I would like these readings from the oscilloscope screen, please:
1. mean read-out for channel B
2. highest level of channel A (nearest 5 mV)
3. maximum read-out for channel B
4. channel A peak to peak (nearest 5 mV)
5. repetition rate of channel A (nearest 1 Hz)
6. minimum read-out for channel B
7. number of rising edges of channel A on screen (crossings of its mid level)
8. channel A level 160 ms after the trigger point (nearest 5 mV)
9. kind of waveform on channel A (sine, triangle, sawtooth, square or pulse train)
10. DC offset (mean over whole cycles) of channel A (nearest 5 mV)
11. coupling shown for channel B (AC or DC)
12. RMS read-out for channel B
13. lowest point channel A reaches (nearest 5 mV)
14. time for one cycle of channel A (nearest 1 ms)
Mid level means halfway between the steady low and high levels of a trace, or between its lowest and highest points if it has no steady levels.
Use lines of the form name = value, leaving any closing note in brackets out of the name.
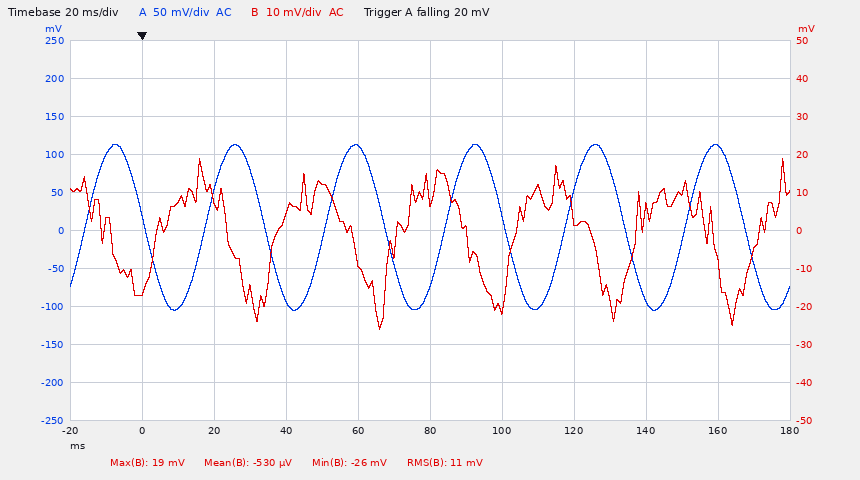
mean read-out for channel B = -530 µV
highest level of channel A = 115 mV
maximum read-out for channel B = 19 mV
channel A peak to peak = 220 mV
repetition rate of channel A = 30 Hz
minimum read-out for channel B = -26 mV
number of rising edges of channel A on screen = 6
channel A level 160 ms after the trigger point = 110 mV
kind of waveform on channel A = sine
DC offset (mean over whole cycles) of channel A = 5 mV
coupling shown for channel B = AC
RMS read-out for channel B = 11 mV
lowest point channel A reaches = -105 mV
time for one cycle of channel A = 33 ms
